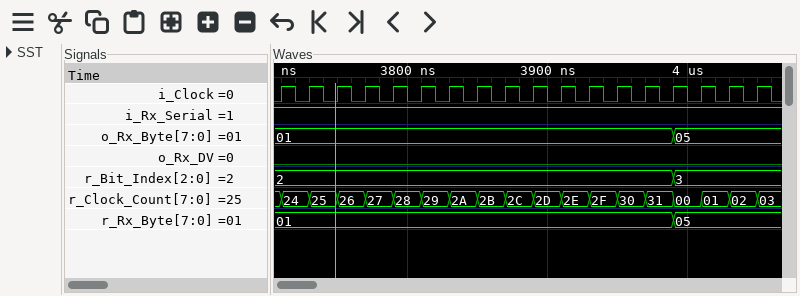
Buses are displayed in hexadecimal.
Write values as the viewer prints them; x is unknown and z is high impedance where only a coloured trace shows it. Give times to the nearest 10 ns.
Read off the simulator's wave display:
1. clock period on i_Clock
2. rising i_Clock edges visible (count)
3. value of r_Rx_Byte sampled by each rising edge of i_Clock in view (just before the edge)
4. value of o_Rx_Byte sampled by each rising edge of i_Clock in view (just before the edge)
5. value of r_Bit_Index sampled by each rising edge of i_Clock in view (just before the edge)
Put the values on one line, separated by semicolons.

20 ns; 18; 01, 01, 01, 01, 01, 01, 01, 01, 01, 01, 01, 01, 01, 01, 01, 05, 05, 05; 01, 01, 01, 01, 01, 01, 01, 01, 01, 01, 01, 01, 01, 01, 01, 05, 05, 05; 2, 2, 2, 2, 2, 2, 2, 2, 2, 2, 2, 2, 2, 2, 2, 3, 3, 3
